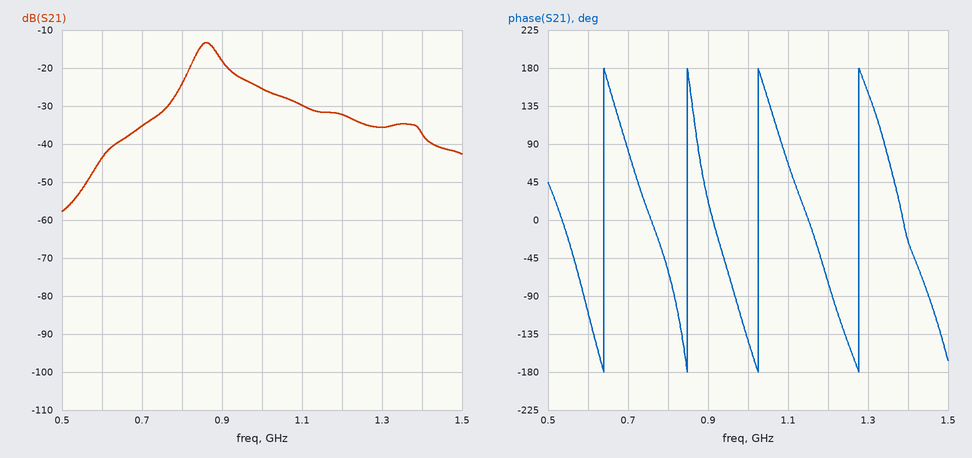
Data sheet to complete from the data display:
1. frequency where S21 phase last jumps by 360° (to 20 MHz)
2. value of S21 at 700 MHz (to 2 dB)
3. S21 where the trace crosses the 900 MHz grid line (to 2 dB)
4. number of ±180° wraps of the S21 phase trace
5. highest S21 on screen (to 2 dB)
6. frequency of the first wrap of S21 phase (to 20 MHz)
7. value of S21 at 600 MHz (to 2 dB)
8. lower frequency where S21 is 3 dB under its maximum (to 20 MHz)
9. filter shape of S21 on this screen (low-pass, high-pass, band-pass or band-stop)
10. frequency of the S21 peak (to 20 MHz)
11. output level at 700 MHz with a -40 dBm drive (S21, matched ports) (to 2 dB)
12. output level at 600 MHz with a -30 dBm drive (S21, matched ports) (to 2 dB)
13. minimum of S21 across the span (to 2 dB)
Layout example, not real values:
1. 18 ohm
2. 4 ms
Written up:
1. 1.28 GHz
2. -36 dB
3. -18 dB
4. 4
5. -14 dB
6. 640 MHz
7. -44 dB
8. 840 MHz
9. band-pass
10. 860 MHz
11. -76 dBm
12. -74 dBm
13. -58 dB
